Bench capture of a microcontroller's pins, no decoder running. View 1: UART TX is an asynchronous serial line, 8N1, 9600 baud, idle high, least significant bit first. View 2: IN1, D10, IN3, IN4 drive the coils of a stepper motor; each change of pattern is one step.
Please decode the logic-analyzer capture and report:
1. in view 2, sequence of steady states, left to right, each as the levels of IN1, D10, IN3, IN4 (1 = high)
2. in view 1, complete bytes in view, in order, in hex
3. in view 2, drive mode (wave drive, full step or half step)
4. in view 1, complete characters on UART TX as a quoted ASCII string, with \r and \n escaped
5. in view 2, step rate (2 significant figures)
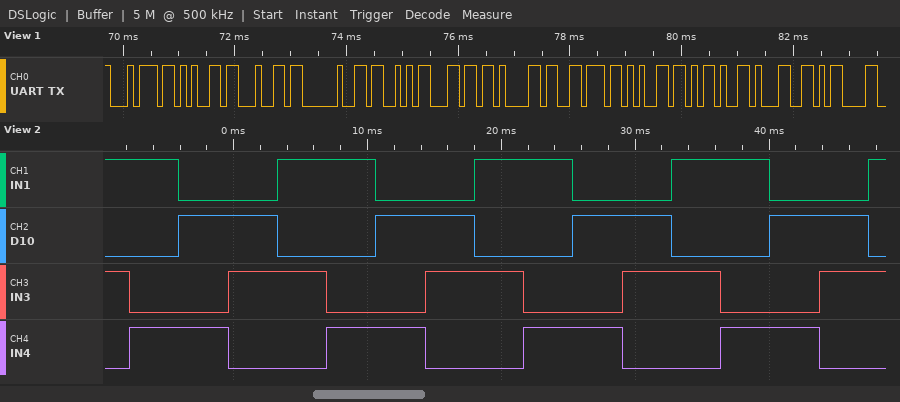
1010 1001 0101 0110 1010 1001 0101 0110 1010 1001 0101 0110 1010 1001 0101 0110 1010
74 65 64 20 53 6C 61 76 65 2D 31 0D
full step
"ted Slave-1\r"
270 steps/s
